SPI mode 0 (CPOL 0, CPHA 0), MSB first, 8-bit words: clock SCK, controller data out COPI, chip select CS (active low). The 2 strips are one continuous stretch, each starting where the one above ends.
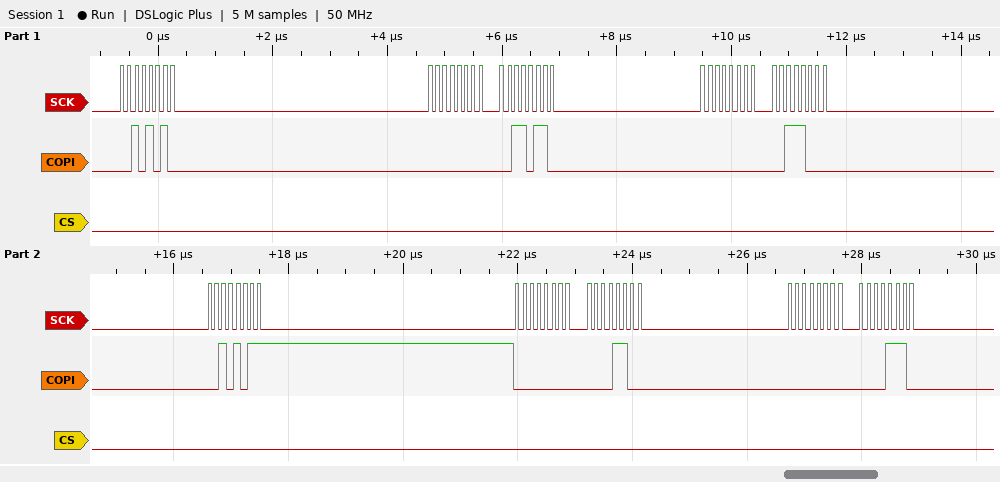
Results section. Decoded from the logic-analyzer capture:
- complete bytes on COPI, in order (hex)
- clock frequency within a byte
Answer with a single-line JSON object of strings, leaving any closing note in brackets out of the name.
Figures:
{"complete bytes on COPI, in order": "2A 00 36 00 38 2B 00 0C 00 0E", "clock frequency within a byte": "8 MHz"}
